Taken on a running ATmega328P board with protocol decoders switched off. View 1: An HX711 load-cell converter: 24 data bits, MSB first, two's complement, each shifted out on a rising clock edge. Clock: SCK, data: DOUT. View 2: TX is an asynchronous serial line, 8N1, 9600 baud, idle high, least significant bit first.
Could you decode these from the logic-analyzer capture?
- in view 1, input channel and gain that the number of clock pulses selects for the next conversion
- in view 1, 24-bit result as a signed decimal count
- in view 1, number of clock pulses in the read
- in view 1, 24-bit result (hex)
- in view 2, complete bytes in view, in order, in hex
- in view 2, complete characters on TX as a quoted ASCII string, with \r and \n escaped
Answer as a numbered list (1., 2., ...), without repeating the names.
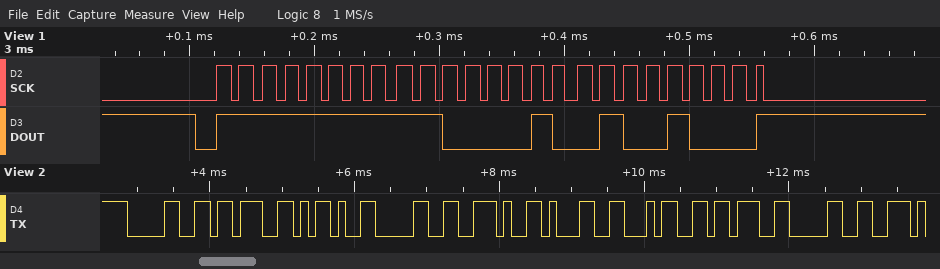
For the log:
1. channel A, gain 128
2. -15800
3. 25
4. 0xFFC248
5. 0x30 0x3B 0x2D 0x30 0x2E 0x31 0x34 0x3B 0x30
6. "0;-0.14;0"
